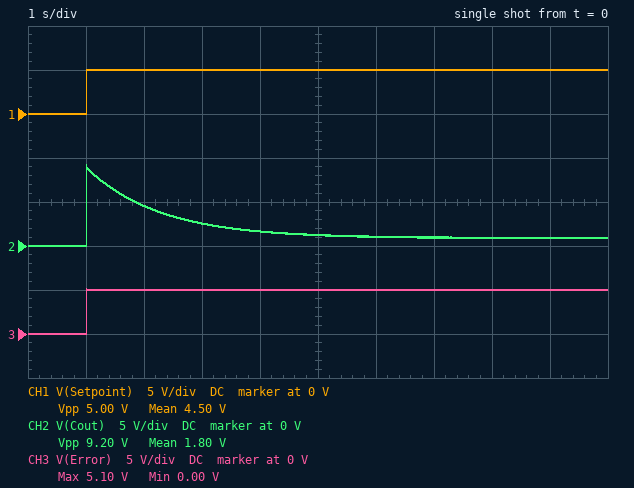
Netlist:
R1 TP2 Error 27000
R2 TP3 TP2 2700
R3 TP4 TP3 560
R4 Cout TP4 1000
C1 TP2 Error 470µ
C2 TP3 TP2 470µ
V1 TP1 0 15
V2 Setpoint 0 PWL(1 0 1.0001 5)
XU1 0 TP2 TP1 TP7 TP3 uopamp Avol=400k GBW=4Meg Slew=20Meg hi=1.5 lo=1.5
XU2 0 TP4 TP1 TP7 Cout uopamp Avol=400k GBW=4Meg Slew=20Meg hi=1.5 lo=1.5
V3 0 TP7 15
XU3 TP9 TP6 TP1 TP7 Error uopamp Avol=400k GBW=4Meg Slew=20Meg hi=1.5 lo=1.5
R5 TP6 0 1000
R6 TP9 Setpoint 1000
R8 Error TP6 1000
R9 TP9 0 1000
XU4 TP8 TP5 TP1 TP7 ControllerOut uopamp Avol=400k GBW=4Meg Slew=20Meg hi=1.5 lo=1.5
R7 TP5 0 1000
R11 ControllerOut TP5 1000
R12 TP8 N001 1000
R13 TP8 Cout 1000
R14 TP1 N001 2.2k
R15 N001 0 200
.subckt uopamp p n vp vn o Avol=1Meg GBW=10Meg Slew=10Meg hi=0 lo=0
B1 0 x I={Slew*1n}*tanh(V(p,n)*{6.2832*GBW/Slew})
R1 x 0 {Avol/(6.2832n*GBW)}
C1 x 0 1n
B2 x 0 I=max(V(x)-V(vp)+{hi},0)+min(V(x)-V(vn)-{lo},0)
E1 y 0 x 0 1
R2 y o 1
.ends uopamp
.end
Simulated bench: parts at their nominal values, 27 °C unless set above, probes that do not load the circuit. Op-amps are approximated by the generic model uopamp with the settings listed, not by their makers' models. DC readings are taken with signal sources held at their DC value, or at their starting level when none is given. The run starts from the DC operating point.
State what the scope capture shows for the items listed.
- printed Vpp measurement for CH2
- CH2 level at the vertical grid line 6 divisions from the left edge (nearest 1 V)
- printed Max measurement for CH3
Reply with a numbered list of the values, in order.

1. 9.20 V
2. 1 V
3. 5.10 V
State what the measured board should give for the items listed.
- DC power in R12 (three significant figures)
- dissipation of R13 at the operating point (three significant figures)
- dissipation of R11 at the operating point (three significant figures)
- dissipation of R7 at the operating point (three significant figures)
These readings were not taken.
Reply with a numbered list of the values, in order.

1. 328 µW
2. 328 µW
3. 328 µW
4. 328 µW
